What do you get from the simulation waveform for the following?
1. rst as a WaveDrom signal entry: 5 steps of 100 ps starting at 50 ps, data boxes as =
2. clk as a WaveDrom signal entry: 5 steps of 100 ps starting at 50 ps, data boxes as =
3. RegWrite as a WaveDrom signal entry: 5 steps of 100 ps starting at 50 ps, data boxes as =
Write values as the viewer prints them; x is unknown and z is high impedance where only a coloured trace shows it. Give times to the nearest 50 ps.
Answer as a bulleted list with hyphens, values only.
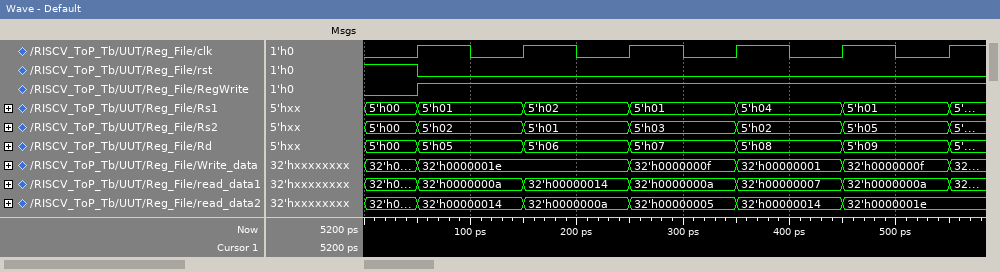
- {name: 'rst', wave: '0....'}
- {name: 'clk', wave: 'p....'}
- {name: 'RegWrite', wave: '1....'}
